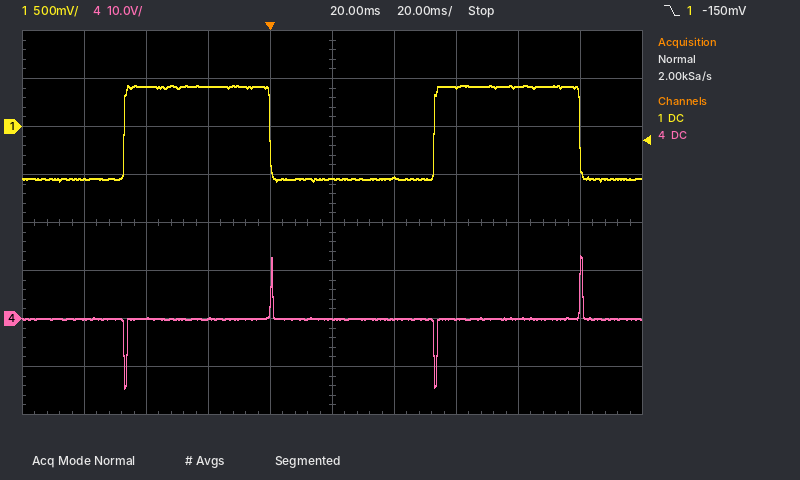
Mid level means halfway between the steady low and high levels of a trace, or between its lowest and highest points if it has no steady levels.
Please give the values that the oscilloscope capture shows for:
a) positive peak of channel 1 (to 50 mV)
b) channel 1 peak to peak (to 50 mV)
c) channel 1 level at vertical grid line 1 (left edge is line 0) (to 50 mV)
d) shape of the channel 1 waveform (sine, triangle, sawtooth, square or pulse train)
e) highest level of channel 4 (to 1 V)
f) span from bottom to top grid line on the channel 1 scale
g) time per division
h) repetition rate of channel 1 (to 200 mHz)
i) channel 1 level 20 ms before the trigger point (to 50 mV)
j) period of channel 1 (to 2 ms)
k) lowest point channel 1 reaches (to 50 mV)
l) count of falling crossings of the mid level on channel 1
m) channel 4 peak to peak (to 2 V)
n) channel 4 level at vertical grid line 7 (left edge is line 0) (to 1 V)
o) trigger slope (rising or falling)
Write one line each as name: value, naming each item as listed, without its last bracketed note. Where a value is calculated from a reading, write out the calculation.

positive peak of channel 1: 450 mV
channel 1 peak to peak: 450 mV − (-550 mV) = 1.00 V
channel 1 level at vertical grid line 1 (left edge is line 0): -550 mV
shape of the channel 1 waveform: square
highest level of channel 4: 13 V
span from bottom to top grid line on the channel 1 scale: 4 V
time per division: 20 ms
repetition rate of channel 1: 1 / 100 ms ≈ 10.0 Hz
channel 1 level 20 ms before the trigger point: 400 mV
period of channel 1: 100 ms
lowest point channel 1 reaches: -550 mV
count of falling crossings of the mid level on channel 1: 2
channel 4 peak to peak: 28 V
channel 4 level at vertical grid line 7 (left edge is line 0): 0 V
trigger slope: falling
